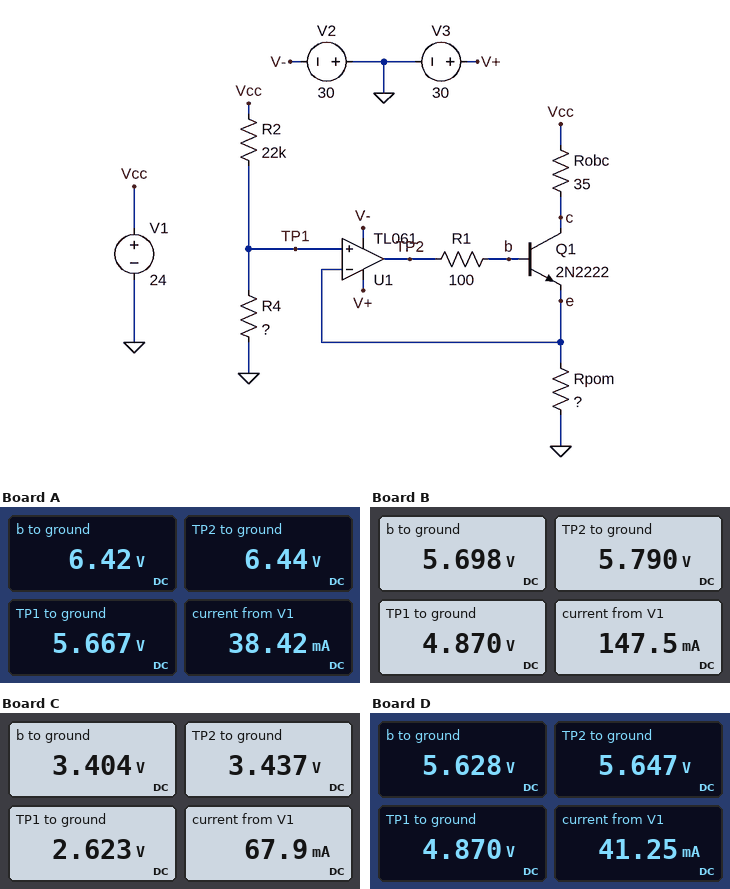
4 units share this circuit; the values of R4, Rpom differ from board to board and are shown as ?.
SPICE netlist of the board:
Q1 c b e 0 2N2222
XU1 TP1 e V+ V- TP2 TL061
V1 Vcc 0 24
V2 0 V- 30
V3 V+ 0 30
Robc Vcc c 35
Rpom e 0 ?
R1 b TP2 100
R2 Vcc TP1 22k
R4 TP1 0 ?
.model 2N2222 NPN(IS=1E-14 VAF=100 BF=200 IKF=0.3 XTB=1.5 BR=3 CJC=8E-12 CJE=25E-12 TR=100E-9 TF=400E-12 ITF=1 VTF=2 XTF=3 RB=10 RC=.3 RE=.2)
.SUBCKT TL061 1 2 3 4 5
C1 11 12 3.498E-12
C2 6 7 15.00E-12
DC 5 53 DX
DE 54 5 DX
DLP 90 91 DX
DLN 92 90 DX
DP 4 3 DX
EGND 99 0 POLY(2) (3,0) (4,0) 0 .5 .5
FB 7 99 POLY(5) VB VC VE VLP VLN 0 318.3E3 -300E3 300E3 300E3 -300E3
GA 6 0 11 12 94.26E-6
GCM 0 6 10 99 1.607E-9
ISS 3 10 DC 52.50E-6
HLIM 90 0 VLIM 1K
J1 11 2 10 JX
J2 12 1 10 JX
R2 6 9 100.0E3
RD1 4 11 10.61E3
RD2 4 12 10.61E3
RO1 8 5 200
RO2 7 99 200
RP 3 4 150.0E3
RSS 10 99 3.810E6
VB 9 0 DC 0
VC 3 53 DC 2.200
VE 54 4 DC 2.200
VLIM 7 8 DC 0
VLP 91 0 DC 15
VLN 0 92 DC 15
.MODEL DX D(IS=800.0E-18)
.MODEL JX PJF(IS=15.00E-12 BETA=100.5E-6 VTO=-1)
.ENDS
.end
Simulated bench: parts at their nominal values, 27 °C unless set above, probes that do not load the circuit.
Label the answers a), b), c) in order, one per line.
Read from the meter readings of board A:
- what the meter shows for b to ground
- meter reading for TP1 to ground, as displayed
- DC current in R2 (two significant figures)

a) 6.42 V
b) 5.667 V
c) 830 µA
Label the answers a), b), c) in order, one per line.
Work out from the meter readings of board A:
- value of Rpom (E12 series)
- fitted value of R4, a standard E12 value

a) 150 Ω
b) 6.8 kΩ
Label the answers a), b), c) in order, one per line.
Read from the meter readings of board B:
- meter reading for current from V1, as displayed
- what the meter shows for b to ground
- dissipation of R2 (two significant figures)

a) 147.5 mA
b) 5.698 V
c) 17 mW
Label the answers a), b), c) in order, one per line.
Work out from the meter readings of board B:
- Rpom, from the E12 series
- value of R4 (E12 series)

a) 33 Ω
b) 5.6 kΩ
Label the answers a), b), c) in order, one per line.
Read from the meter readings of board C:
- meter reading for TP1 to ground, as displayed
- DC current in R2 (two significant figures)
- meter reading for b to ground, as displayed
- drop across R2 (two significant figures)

a) 2.623 V
b) 970 µA
c) 3.404 V
d) 21 V
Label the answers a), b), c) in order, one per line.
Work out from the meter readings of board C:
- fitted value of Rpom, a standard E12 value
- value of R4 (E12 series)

a) 39 Ω
b) 2.7 kΩ
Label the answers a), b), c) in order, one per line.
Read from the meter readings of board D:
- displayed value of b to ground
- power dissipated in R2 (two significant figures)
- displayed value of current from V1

a) 5.628 V
b) 17 mW
c) 41.25 mA
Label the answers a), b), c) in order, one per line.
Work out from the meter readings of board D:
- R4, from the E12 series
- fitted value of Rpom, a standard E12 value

a) 5.6 kΩ
b) 120 Ω
